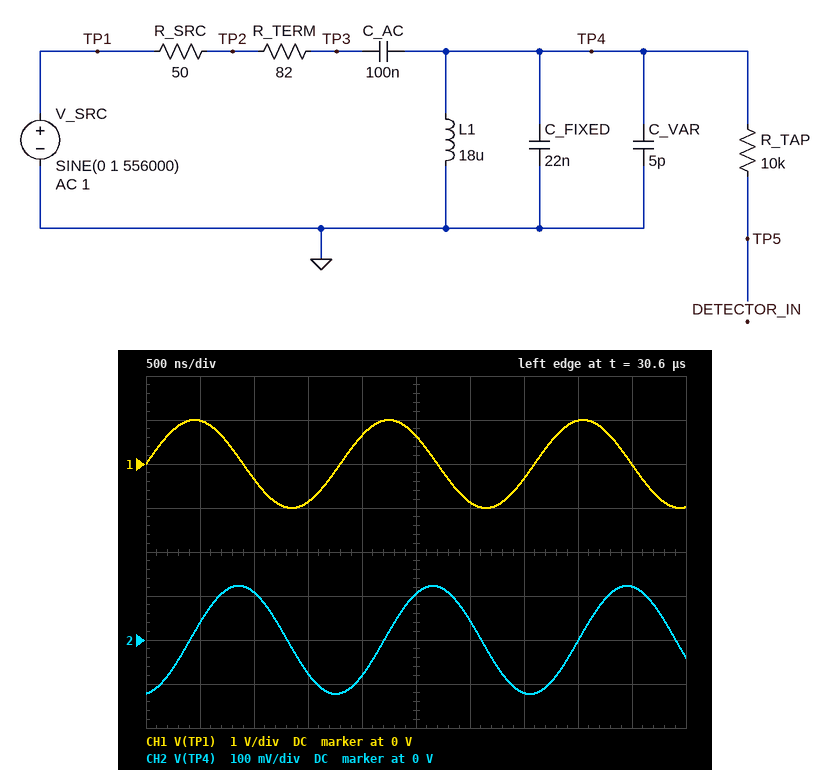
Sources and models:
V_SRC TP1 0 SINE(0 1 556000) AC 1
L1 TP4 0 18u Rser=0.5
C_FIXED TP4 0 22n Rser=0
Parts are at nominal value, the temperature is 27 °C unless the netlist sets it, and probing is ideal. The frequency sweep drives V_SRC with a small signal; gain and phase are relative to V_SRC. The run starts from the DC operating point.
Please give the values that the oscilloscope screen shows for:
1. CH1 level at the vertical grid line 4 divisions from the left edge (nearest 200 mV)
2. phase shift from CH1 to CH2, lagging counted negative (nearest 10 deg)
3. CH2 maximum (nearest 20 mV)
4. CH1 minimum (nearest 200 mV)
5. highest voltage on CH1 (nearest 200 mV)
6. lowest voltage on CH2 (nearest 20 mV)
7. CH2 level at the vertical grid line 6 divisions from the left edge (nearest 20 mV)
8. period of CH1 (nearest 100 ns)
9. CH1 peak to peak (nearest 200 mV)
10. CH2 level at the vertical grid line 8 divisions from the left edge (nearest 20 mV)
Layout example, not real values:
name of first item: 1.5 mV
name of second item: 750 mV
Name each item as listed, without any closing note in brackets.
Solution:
CH1 level at the vertical grid line 4 divisions from the left edge: 600 mV
phase shift from CH1 to CH2, lagging counted negative: -80 deg
CH2 maximum: 120 mV
CH1 minimum: -1.0 V
highest voltage on CH1: 1.0 V
lowest voltage on CH2: -120 mV
CH2 level at the vertical grid line 6 divisions from the left edge: 40 mV
period of CH1: 1.8 µs
CH1 peak to peak: 2.0 V
CH2 level at the vertical grid line 8 divisions from the left edge: 0 V
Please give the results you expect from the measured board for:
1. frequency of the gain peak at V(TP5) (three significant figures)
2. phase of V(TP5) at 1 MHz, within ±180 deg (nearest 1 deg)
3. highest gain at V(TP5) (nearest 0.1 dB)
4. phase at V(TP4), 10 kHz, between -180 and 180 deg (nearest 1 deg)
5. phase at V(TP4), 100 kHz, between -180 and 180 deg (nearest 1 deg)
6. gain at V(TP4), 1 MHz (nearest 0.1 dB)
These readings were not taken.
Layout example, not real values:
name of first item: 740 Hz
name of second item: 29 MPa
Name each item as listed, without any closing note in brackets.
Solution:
frequency of the gain peak at V(TP5): 252 kHz
phase of V(TP5) at 1 MHz, within ±180 deg: -86 deg
highest gain at V(TP5): -0.7 dB
phase at V(TP4), 10 kHz, between -180 and 180 deg: 116 deg
phase at V(TP4), 100 kHz, between -180 and 180 deg: 88 deg
gain at V(TP4), 1 MHz: -24.7 dB
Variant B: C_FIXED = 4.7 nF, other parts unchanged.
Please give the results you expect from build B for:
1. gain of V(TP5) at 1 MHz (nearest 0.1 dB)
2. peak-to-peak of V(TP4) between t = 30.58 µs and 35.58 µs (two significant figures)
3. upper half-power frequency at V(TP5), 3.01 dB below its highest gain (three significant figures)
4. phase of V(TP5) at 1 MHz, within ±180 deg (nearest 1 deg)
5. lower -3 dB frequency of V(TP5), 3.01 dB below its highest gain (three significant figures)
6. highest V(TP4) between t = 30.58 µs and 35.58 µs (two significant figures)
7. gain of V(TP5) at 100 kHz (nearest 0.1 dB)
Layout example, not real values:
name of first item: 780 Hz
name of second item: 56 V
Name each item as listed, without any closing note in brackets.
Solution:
gain of V(TP5) at 1 MHz: -9.3 dB
peak-to-peak of V(TP4) between t = 30.58 µs and 35.58 µs: 2.0 V
upper half-power frequency at V(TP5), 3.01 dB below its highest gain: 691 kHz
phase of V(TP5) at 1 MHz, within ±180 deg: -69 deg
lower -3 dB frequency of V(TP5), 3.01 dB below its highest gain: 430 kHz
highest V(TP4) between t = 30.58 µs and 35.58 µs: 980 mV
gain of V(TP5) at 100 kHz: -21.1 dB
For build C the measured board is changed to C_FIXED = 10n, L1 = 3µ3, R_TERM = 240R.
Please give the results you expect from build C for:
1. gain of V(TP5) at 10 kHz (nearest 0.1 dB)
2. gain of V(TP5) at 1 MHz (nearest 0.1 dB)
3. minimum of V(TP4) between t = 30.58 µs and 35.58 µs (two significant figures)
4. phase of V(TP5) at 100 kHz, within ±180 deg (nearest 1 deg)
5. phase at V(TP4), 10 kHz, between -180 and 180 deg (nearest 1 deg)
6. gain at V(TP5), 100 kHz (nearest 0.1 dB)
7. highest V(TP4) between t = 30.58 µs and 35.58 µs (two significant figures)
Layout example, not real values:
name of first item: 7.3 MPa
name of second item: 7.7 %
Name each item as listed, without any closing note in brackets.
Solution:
gain of V(TP5) at 10 kHz: -55.7 dB
gain of V(TP5) at 1 MHz: -13.0 dB
minimum of V(TP4) between t = 30.58 µs and 35.58 µs: -66 mV
phase of V(TP5) at 100 kHz, within ±180 deg: 79 deg
phase at V(TP4), 10 kHz, between -180 and 180 deg: 51 deg
gain at V(TP5), 100 kHz: -42.6 dB
highest V(TP4) between t = 30.58 µs and 35.58 µs: 66 mV
